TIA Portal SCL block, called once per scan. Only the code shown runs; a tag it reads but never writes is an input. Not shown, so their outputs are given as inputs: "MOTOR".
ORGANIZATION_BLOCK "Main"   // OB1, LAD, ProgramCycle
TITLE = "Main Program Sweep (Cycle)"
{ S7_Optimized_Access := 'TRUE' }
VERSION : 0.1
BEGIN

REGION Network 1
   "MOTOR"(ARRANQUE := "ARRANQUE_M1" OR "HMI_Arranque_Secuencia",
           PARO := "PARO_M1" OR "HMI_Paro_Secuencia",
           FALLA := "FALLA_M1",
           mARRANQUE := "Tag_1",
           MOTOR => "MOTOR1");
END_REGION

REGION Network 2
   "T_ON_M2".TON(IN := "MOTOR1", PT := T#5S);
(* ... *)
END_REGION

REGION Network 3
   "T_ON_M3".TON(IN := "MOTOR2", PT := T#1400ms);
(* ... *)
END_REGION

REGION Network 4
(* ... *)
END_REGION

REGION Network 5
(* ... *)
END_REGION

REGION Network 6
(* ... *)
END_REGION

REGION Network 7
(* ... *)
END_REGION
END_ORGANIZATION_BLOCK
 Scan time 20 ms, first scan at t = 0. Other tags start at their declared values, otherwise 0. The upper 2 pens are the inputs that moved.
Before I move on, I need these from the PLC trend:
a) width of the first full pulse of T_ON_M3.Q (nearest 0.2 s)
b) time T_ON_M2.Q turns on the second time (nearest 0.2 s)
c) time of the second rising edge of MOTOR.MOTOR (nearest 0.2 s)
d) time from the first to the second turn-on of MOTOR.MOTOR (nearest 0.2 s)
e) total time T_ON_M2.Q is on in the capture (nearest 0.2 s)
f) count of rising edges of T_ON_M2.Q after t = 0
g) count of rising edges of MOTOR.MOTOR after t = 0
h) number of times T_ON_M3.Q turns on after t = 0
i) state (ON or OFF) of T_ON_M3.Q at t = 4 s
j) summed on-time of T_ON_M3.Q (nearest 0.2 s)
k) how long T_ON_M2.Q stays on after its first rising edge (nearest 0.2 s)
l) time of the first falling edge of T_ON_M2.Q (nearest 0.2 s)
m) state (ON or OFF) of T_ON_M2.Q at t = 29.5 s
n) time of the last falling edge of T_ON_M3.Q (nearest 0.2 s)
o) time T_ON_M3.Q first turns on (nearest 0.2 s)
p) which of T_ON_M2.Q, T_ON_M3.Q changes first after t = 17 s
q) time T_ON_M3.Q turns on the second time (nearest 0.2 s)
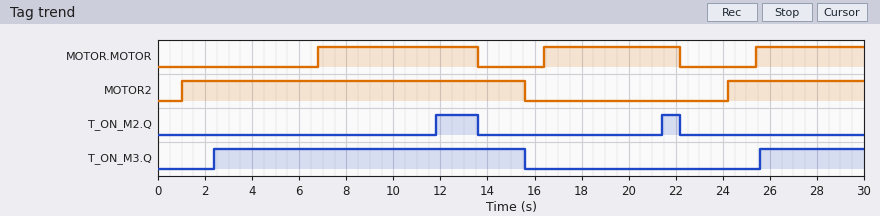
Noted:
13.2 s
21.4 s
16.4 s
9.6 s
2.6 s
2
3
2
ON
17.6 s
1.8 s
13.6 s
OFF
15.6 s
2.4 s
T_ON_M2.Q
25.6 s
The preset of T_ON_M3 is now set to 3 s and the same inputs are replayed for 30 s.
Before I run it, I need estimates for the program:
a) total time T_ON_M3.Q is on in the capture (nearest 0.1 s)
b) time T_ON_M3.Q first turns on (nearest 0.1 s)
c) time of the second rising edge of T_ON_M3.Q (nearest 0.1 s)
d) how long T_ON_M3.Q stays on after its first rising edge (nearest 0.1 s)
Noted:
14.4 s
4.0 s
27.2 s
11.6 s
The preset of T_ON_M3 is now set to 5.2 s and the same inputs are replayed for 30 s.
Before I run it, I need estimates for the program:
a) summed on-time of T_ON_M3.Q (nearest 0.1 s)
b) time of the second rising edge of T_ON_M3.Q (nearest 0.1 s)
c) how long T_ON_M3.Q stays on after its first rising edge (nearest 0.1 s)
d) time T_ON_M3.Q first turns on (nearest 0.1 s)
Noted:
10.0 s
29.4 s
9.4 s
6.2 s
